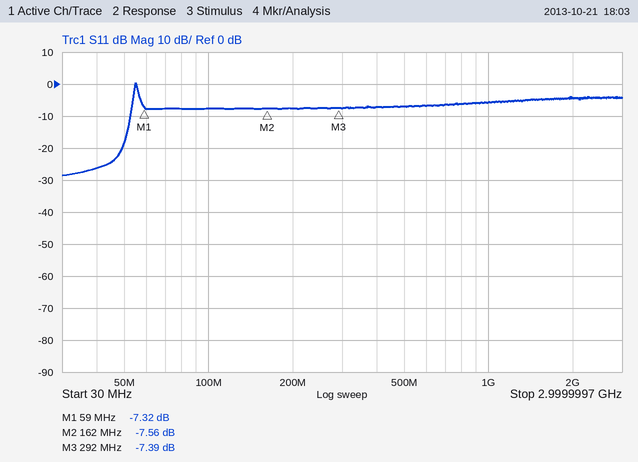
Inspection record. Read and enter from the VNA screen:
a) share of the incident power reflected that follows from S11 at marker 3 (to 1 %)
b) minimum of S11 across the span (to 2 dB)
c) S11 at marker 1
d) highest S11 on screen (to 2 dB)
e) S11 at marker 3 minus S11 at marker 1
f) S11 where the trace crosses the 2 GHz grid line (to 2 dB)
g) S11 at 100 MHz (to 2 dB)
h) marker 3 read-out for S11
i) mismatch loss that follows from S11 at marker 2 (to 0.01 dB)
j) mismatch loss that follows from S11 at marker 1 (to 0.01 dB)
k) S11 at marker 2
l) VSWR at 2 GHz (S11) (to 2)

18 %
-28 dB
-7.32 dB
0 dB
-0.07 dB
-4 dB
-8 dB
-7.39 dB
0.84 dB
0.89 dB
-7.56 dB
4
